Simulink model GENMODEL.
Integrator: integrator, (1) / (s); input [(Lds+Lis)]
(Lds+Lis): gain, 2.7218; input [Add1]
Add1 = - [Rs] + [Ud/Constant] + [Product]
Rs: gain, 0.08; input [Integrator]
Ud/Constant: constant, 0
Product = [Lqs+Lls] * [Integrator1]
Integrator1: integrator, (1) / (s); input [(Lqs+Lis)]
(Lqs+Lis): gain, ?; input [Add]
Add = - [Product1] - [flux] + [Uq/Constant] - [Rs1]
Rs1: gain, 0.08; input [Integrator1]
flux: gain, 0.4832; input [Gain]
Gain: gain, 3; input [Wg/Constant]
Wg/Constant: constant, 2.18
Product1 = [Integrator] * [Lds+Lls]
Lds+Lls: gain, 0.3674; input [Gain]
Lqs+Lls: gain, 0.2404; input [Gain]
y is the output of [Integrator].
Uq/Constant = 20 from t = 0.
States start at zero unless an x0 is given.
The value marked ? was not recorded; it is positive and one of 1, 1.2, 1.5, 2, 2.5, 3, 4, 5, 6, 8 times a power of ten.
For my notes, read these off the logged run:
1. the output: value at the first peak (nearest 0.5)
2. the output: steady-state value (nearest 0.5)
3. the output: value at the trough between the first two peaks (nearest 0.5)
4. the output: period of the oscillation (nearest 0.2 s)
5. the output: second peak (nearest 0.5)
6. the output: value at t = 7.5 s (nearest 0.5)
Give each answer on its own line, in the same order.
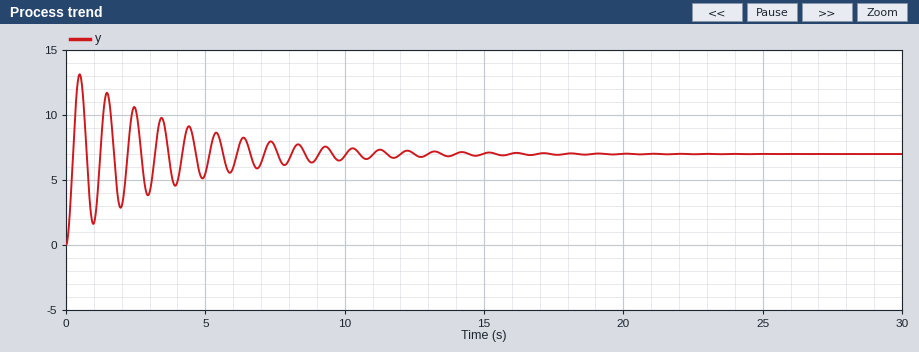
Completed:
13.0
7.0
1.5
1.0 s
11.5
7.5
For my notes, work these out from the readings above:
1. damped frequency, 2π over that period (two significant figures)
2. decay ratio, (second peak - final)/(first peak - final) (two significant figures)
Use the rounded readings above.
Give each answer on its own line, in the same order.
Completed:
6.3 rad/s
0.75
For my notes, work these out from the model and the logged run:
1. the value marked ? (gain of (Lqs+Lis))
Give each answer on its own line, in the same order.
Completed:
4
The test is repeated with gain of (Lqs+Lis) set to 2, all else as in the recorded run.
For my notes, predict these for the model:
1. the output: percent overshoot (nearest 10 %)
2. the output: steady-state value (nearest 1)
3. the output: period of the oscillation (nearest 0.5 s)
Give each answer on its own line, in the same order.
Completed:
90 %
7
1.5 s
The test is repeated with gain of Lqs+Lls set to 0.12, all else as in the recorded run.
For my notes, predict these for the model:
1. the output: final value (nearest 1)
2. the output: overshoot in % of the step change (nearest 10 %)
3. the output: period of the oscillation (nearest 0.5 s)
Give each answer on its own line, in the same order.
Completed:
7
80 %
1.5 s
